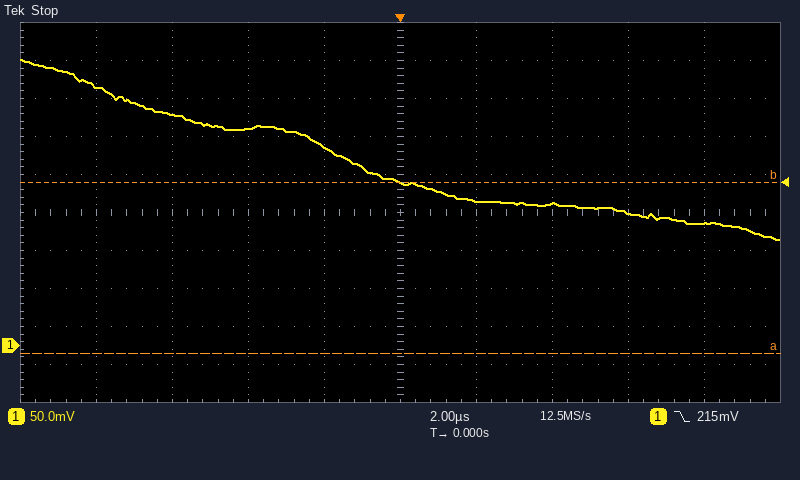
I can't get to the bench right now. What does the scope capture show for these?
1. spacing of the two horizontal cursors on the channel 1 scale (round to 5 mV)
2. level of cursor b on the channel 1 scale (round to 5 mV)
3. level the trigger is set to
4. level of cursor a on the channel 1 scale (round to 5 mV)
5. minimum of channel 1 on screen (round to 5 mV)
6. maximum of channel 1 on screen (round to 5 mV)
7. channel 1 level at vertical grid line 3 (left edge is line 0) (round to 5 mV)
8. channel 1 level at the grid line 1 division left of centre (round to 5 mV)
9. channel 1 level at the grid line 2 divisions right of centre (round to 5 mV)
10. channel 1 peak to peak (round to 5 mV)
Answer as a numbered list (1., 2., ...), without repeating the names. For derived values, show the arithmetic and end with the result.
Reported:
1. 225 mV
2. 215 mV
3. 215 mV
4. -10 mV
5. 140 mV
6. 375 mV
7. 285 mV
8. 260 mV
9. 185 mV
10. 375 mV − (140 mV) = 235 mV
